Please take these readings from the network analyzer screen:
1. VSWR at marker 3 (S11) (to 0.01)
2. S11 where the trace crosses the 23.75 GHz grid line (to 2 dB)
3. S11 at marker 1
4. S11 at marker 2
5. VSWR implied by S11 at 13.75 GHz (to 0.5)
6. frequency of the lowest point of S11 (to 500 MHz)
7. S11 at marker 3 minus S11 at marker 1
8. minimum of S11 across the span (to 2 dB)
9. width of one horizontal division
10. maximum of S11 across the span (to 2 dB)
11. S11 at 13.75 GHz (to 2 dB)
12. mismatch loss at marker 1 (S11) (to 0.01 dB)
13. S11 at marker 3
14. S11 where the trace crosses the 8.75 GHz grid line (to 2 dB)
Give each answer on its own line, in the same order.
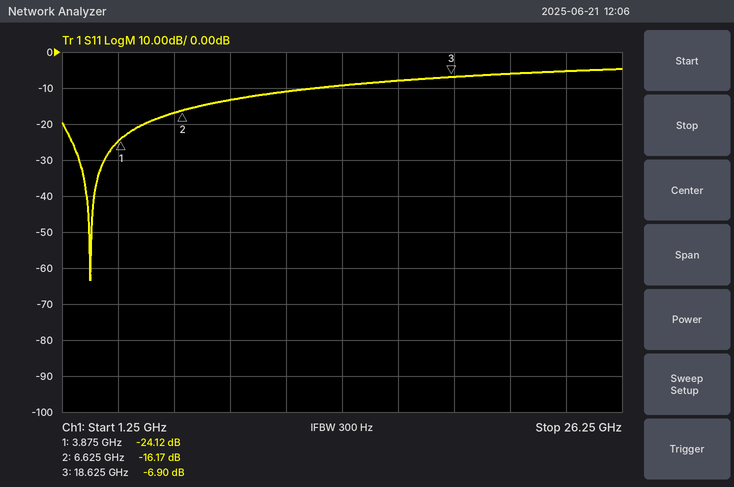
2.65
-6 dB
-24.12 dB
-16.17 dB
2.0
2.5 GHz
17.22 dB
-64 dB
2.5 GHz
-4 dB
-10 dB
0.02 dB
-6.90 dB
-14 dB
